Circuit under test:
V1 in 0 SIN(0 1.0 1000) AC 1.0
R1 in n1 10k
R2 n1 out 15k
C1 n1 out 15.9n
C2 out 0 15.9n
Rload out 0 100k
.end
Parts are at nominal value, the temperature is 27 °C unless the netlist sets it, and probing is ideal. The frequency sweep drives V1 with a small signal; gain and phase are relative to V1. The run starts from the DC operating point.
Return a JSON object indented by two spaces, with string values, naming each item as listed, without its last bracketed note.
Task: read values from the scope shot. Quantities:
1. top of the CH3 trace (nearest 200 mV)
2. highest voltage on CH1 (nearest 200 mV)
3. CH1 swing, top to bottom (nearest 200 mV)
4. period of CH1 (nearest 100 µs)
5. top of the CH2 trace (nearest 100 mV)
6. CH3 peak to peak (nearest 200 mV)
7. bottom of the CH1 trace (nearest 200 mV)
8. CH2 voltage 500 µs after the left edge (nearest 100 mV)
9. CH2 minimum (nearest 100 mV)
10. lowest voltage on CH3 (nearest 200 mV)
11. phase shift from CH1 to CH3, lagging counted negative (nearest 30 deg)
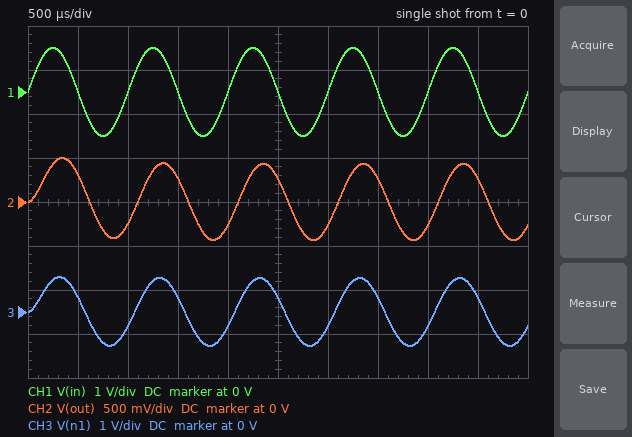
{
  "top of the CH3 trace": "800 mV",
  "highest voltage on CH1": "1.0 V",
  "CH1 swing, top to bottom": "2.0 V",
  "period of CH1": "1.0 ms",
  "top of the CH2 trace": "500 mV",
  "CH3 peak to peak": "1.6 V",
  "bottom of the CH1 trace": "-1.0 V",
  "CH2 voltage 500 µs after the left edge": "300 mV",
  "CH2 minimum": "-400 mV",
  "lowest voltage on CH3": "-800 mV",
  "phase shift from CH1 to CH3, lagging counted negative": "-30 deg"
}
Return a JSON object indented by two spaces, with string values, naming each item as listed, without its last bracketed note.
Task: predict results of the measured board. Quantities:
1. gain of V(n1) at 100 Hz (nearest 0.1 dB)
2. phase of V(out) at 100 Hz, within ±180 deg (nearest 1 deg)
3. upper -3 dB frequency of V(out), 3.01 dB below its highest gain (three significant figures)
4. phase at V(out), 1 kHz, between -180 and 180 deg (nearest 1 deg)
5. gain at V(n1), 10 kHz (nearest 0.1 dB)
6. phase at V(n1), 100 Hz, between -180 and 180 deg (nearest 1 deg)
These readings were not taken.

{
  "gain of V(n1) at 100 Hz": "-0.8 dB",
  "phase of V(out) at 100 Hz, within ±180 deg": "-10 deg",
  "upper -3 dB frequency of V(out), 3.01 dB below its highest gain": "475 Hz",
  "phase at V(out), 1 kHz, between -180 and 180 deg": "-37 deg",
  "gain at V(n1), 10 kHz": "-14.2 dB",
  "phase at V(n1), 100 Hz, between -180 and 180 deg": "-4 deg"
}
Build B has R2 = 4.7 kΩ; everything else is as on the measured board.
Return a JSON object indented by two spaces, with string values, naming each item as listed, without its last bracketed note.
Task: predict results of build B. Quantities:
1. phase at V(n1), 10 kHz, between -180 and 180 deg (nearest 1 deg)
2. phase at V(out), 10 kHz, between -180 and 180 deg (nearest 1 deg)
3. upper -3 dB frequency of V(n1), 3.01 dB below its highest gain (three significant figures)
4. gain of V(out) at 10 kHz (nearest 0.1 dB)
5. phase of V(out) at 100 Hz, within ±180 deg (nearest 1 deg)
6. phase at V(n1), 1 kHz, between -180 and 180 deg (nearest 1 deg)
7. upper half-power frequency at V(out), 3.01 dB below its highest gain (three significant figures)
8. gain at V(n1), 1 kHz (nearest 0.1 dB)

{
  "phase at V(n1), 10 kHz, between -180 and 180 deg": "-73 deg",
  "phase at V(out), 10 kHz, between -180 and 180 deg": "-79 deg",
  "upper -3 dB frequency of V(n1), 3.01 dB below its highest gain": "1.13 kHz",
  "gain of V(out) at 10 kHz": "-20.3 dB",
  "phase of V(out) at 100 Hz, within ±180 deg": "-7 deg",
  "phase at V(n1), 1 kHz, between -180 and 180 deg": "-29 deg",
  "upper half-power frequency at V(out), 3.01 dB below its highest gain": "740 Hz",
  "gain at V(n1), 1 kHz": "-3.5 dB"
}
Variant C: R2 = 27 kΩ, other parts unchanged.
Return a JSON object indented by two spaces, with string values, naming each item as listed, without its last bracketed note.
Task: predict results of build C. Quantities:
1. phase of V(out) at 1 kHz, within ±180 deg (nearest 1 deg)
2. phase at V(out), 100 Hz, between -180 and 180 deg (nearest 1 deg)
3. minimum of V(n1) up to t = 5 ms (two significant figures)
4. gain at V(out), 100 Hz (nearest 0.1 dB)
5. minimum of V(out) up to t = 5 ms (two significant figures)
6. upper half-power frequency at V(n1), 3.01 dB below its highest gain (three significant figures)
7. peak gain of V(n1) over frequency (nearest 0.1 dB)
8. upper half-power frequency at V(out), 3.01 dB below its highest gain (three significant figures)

{
  "phase of V(out) at 1 kHz, within ±180 deg": "-32 deg",
  "phase at V(out), 100 Hz, between -180 and 180 deg": "-11 deg",
  "minimum of V(n1) up to t = 5 ms": "-820 mV",
  "gain at V(out), 100 Hz": "-3.2 dB",
  "minimum of V(out) up to t = 5 ms": "-420 mV",
  "upper half-power frequency at V(n1), 3.01 dB below its highest gain": "2.07 kHz",
  "peak gain of V(n1) over frequency": "-0.7 dB",
  "upper half-power frequency at V(out), 3.01 dB below its highest gain": "414 Hz"
}
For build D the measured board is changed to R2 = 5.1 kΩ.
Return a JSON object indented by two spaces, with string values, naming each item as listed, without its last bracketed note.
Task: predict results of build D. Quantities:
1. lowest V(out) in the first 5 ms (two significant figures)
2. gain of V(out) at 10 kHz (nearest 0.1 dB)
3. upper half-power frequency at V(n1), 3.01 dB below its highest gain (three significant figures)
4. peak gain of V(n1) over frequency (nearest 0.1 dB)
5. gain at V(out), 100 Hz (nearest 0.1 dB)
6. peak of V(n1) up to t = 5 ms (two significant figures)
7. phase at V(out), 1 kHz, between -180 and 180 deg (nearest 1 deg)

{
  "lowest V(out) in the first 5 ms": "-520 mV",
  "gain of V(out) at 10 kHz": "-20.3 dB",
  "upper half-power frequency at V(n1), 3.01 dB below its highest gain": "1.17 kHz",
  "peak gain of V(n1) over frequency": "-0.8 dB",
  "gain at V(out), 100 Hz": "-1.3 dB",
  "peak of V(n1) up to t = 5 ms": "720 mV",
  "phase at V(out), 1 kHz, between -180 and 180 deg": "-46 deg"
}
